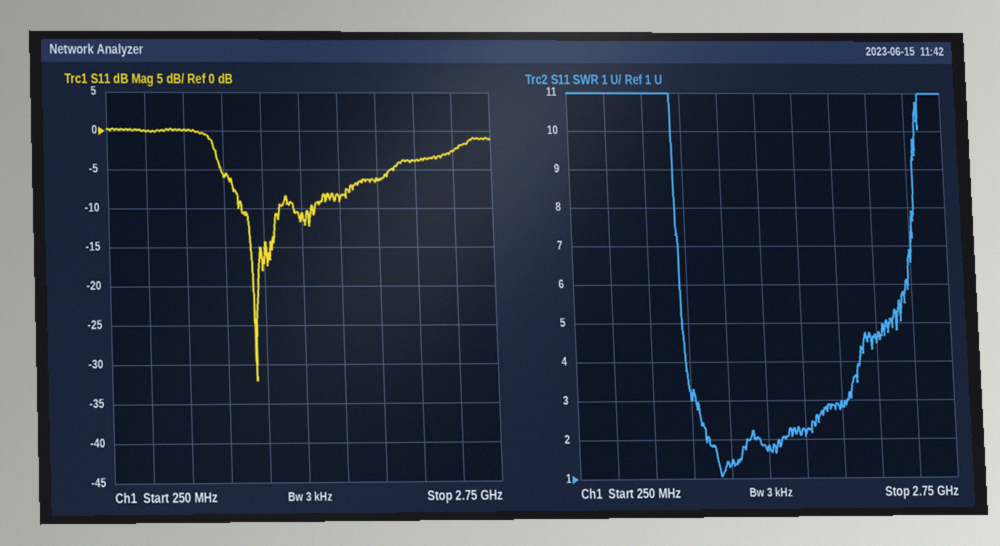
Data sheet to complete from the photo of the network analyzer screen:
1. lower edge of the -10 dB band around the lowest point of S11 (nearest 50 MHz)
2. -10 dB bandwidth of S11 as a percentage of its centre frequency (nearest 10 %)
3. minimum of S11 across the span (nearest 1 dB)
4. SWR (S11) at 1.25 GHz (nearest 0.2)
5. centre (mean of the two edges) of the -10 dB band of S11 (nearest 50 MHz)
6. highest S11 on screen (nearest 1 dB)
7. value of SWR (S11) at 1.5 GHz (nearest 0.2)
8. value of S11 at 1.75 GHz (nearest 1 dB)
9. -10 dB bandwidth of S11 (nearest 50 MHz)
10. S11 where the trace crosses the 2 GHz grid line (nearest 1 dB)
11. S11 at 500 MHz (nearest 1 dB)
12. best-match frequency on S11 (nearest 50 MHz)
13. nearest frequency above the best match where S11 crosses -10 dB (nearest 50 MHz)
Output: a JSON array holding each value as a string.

["1.10 GHz", "20 %", "-32 dB", "1.4", "1.25 GHz", "0 dB", "1.8", "-9 dB", "250 MHz", "-6 dB", "0 dB", "1.20 GHz", "1.35 GHz"]
